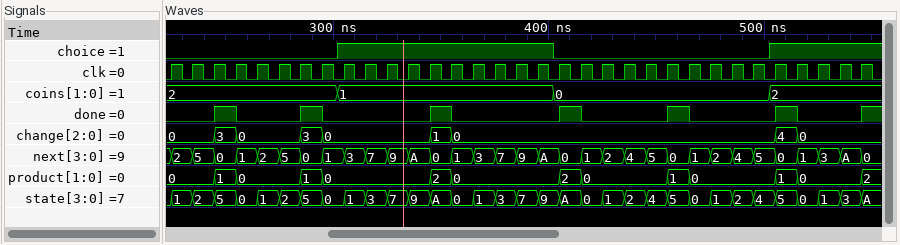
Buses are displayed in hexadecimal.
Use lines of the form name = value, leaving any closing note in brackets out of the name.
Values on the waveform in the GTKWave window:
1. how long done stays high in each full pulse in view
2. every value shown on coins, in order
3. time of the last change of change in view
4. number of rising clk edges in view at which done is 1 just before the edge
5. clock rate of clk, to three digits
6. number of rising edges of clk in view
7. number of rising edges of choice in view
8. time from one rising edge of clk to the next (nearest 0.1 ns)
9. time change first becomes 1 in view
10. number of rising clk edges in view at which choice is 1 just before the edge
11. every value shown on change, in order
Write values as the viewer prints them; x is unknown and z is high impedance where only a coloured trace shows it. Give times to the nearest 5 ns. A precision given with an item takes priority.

how long done stays high in each full pulse in view = 10 ns, 10 ns, 10 ns, 10 ns, 10 ns, 10 ns
every value shown on coins, in order = 2, 1, 0, 2
time of the last change of change in view = 515 ns
number of rising clk edges in view at which done is 1 just before the edge = 6
clock rate of clk, to three digits = 100 MHz
number of rising edges of clk in view = 33
number of rising edges of choice in view = 2
time from one rising edge of clk to the next = 10 ns
time change first becomes 1 in view = 345 ns
number of rising clk edges in view at which choice is 1 just before the edge = 15
every value shown on change, in order = 0, 3, 0, 3, 0, 1, 0, 4, 0
